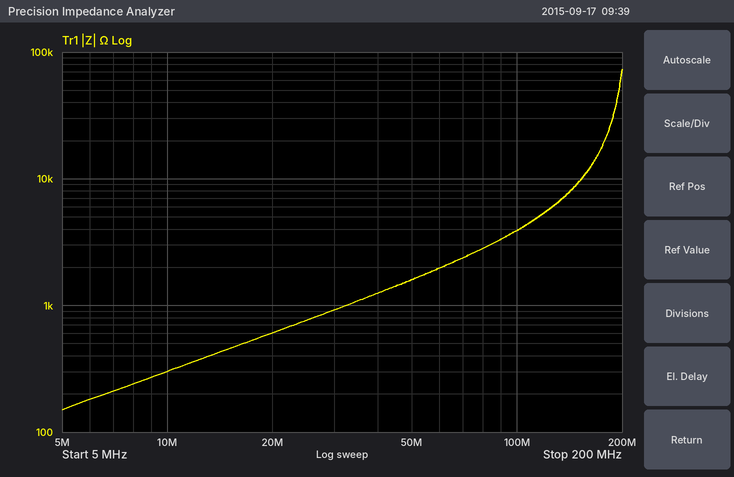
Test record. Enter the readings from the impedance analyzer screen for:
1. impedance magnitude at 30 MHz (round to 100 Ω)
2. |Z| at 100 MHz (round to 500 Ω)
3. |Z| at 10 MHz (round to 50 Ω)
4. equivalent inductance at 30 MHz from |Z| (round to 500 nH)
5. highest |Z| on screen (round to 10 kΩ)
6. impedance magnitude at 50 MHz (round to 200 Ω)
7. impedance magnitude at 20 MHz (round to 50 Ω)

900 Ω
4.0 kΩ
300 Ω
5.0 µH
70 kΩ
1.6 kΩ
600 Ω
